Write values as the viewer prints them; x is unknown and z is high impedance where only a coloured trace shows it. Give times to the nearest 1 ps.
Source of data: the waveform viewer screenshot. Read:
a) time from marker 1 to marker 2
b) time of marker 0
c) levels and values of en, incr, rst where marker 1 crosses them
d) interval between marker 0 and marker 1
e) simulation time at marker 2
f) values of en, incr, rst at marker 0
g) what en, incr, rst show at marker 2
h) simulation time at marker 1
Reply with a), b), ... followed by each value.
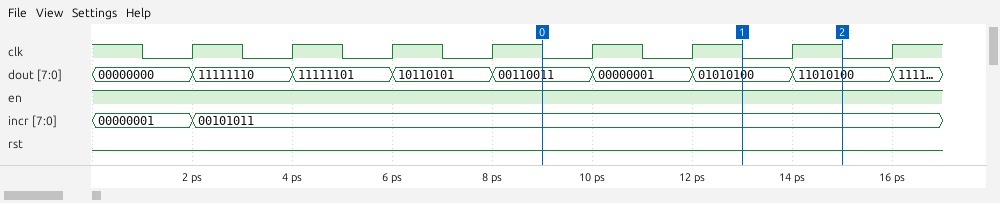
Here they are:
a) 2 ps
b) 9 ps
c) en=1, incr=00101011, rst=0
d) 4 ps
e) 15 ps
f) en=1, incr=00101011, rst=0
g) en=1, incr=00101011, rst=0
h) 13 ps
